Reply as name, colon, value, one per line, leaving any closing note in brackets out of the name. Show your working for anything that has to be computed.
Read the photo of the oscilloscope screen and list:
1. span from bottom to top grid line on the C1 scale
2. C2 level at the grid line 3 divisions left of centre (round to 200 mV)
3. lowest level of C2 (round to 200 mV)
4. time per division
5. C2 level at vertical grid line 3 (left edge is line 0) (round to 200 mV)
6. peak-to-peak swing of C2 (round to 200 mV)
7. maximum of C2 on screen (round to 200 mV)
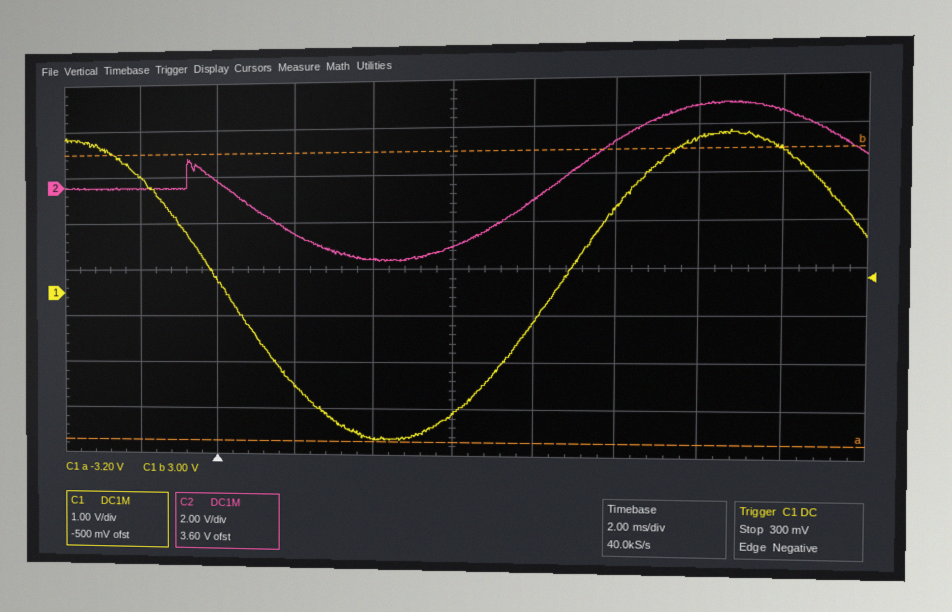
span from bottom to top grid line on the C1 scale: 8 V
C2 level at the grid line 3 divisions left of centre: 200 mV
lowest level of C2: -3.2 V
time per division: 2 ms
C2 level at vertical grid line 3 (left edge is line 0): -2.0 V
peak-to-peak swing of C2: 3.4 V − (-3.2 V) = 6.6 V
maximum of C2 on screen: 3.4 V
